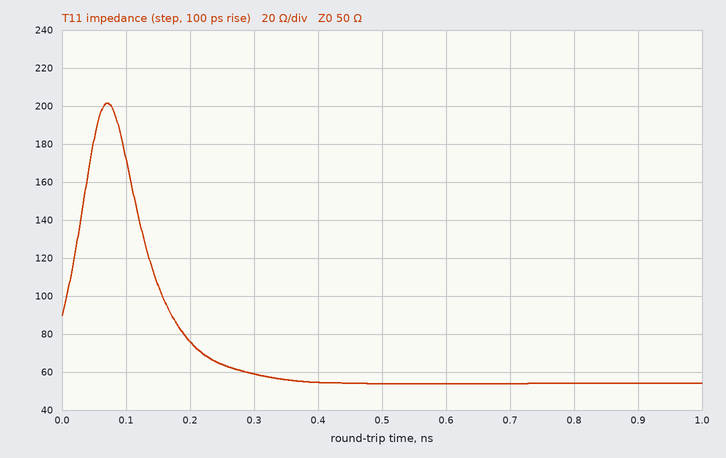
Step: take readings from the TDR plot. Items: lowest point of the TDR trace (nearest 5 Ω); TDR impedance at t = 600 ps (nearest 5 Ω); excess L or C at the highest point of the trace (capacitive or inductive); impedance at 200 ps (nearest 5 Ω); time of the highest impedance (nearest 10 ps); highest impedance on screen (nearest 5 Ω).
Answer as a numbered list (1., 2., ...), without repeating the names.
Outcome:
1. 55 Ω
2. 55 Ω
3. inductive
4. 75 Ω
5. 70 ps
6. 200 Ω
